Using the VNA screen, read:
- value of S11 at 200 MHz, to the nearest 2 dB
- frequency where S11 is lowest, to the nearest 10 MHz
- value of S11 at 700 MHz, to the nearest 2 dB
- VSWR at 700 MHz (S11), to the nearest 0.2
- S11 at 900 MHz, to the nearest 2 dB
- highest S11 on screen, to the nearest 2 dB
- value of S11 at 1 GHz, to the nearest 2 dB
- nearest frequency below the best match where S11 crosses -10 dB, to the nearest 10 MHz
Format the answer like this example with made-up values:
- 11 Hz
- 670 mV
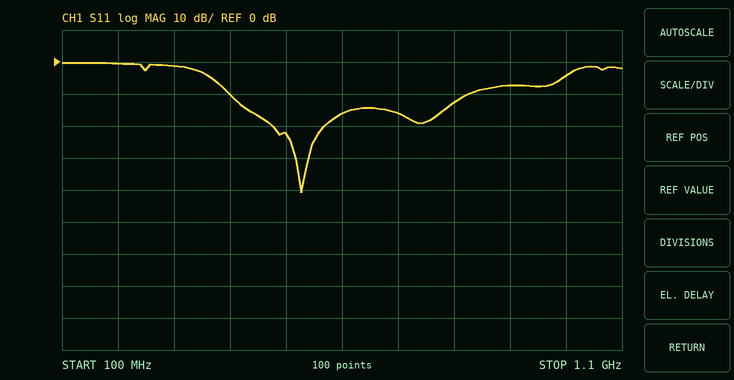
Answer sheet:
- 0 dB
- 530 MHz
- -16 dB
- 1.4
- -8 dB
- 0 dB
- -4 dB
- 400 MHz
